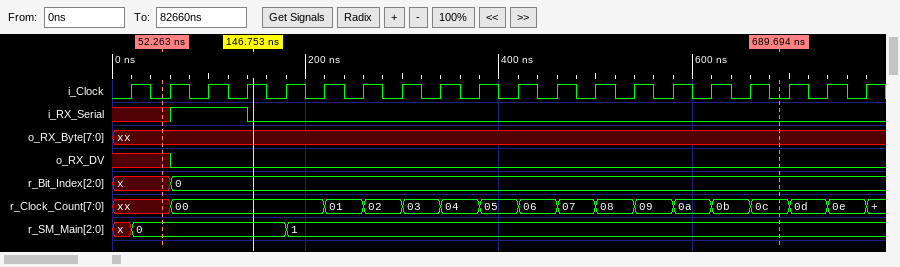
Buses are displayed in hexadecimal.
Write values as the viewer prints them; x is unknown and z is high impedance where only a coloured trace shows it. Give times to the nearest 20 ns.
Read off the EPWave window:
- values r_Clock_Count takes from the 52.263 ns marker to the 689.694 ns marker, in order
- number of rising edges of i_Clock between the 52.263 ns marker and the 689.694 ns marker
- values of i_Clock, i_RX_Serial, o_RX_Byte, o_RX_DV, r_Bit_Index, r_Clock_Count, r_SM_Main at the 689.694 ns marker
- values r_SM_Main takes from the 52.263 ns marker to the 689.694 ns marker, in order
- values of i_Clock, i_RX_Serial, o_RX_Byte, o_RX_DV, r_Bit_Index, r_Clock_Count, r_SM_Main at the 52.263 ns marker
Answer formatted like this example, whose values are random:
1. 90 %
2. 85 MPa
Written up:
1. xx, 00, 01, 02, 03, 04, 05, 06, 07, 08, 09, 0a, 0b, 0c
2. 16
3. i_Clock=0, i_RX_Serial=0, o_RX_Byte=xx, o_RX_DV=0, r_Bit_Index=0, r_Clock_Count=0c, r_SM_Main=1
4. 0, 1
5. i_Clock=0, i_RX_Serial=x, o_RX_Byte=xx, o_RX_DV=x, r_Bit_Index=x, r_Clock_Count=xx, r_SM_Main=0
